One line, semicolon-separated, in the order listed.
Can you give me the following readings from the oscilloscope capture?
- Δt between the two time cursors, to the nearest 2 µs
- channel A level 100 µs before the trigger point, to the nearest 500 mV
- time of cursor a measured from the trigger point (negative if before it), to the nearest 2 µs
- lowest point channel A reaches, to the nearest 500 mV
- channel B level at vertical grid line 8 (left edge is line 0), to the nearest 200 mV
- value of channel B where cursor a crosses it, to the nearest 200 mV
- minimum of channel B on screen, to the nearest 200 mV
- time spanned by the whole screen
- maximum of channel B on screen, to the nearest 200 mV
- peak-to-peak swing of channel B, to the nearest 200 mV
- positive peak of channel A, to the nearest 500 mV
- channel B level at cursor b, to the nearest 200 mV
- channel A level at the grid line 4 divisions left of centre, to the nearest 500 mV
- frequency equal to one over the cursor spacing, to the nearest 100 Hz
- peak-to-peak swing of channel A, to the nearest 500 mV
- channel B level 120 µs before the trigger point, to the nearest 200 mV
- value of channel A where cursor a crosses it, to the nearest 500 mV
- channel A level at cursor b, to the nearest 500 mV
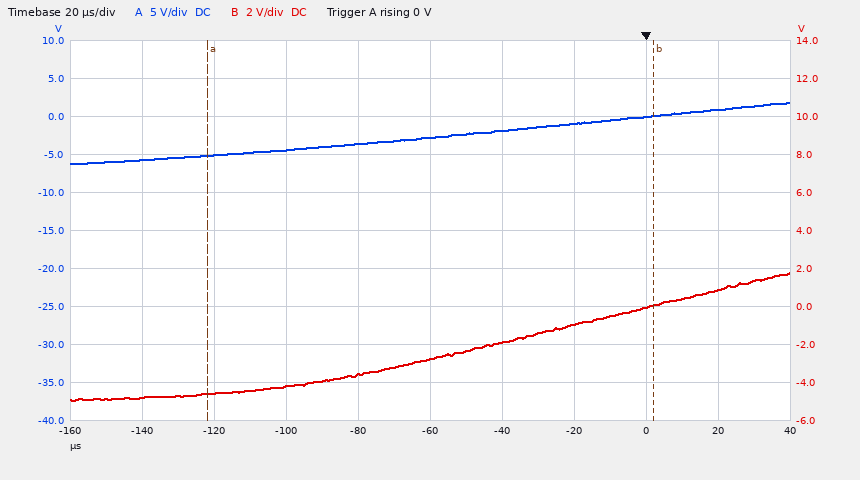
124 µs; -4.5 V; -122 µs; -6.0 V; 0.0 V; -4.6 V; -5.0 V; 200 µs; 1.8 V; 6.8 V; 2.0 V; 0.0 V; -5.5 V; 8.1 kHz; 8.0 V; -4.6 V; -5.0 V; 0.0 V
